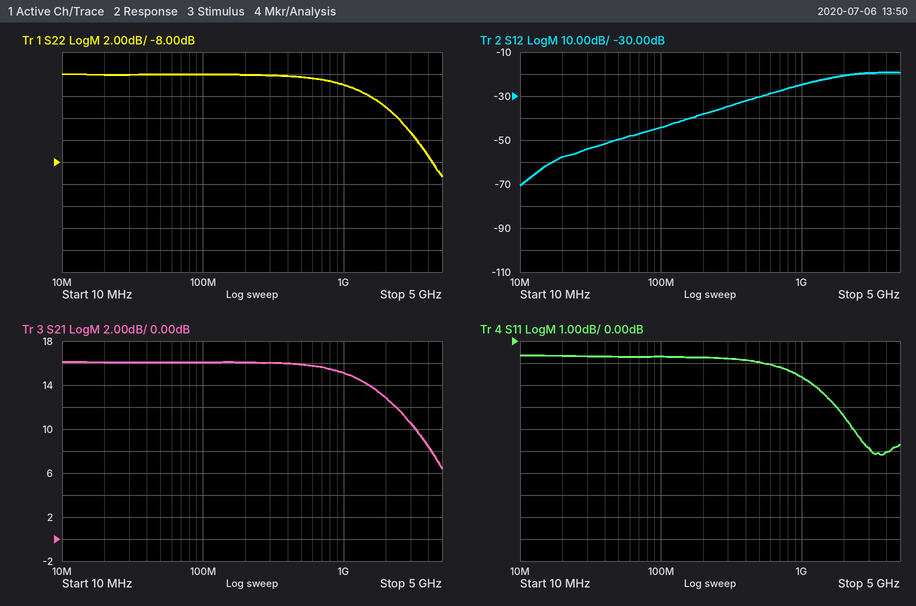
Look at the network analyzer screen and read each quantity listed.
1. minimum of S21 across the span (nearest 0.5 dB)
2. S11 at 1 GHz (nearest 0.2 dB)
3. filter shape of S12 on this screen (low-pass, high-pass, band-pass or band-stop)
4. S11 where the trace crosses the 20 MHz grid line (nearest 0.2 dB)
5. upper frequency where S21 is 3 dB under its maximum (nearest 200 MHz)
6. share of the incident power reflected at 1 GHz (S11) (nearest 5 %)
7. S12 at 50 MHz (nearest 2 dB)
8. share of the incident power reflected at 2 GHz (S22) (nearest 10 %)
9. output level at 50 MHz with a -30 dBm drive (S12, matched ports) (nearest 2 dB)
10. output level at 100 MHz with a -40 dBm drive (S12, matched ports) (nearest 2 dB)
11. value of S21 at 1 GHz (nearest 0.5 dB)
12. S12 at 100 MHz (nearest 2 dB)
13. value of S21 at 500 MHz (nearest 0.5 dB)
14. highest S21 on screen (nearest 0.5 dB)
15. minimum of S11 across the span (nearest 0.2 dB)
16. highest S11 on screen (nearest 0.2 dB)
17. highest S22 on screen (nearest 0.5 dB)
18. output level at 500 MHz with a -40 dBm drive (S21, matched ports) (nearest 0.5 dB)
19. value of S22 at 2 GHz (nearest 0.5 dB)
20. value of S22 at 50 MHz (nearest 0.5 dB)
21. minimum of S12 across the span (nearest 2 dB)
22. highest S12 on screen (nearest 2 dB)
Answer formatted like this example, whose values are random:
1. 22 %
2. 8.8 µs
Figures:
1. 6.5 dB
2. -1.6 dB
3. high-pass
4. -0.6 dB
5. 1.8 GHz
6. 70 %
7. -50 dB
8. 50 %
9. -80 dBm
10. -84 dBm
11. 15.0 dB
12. -44 dB
13. 16.0 dB
14. 16.0 dB
15. -5.2 dB
16. -0.6 dB
17. 0.0 dB
18. -24.0 dBm
19. -3.0 dB
20. 0.0 dB
21. -70 dB
22. -20 dB
